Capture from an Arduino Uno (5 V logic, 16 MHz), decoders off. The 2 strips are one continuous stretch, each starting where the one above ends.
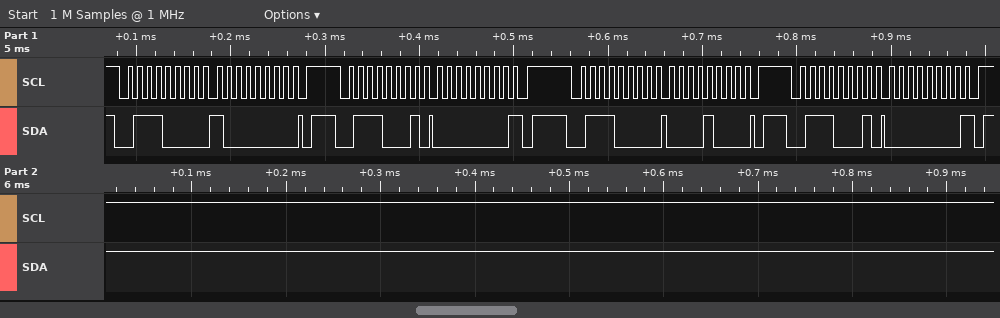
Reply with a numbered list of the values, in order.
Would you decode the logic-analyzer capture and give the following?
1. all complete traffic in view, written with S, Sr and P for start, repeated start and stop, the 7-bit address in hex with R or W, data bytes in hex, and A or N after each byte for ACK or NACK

1. S 38W A 80 A P S 38R A 00 N P S 38W A 08 A P S 38R A 00 N P
